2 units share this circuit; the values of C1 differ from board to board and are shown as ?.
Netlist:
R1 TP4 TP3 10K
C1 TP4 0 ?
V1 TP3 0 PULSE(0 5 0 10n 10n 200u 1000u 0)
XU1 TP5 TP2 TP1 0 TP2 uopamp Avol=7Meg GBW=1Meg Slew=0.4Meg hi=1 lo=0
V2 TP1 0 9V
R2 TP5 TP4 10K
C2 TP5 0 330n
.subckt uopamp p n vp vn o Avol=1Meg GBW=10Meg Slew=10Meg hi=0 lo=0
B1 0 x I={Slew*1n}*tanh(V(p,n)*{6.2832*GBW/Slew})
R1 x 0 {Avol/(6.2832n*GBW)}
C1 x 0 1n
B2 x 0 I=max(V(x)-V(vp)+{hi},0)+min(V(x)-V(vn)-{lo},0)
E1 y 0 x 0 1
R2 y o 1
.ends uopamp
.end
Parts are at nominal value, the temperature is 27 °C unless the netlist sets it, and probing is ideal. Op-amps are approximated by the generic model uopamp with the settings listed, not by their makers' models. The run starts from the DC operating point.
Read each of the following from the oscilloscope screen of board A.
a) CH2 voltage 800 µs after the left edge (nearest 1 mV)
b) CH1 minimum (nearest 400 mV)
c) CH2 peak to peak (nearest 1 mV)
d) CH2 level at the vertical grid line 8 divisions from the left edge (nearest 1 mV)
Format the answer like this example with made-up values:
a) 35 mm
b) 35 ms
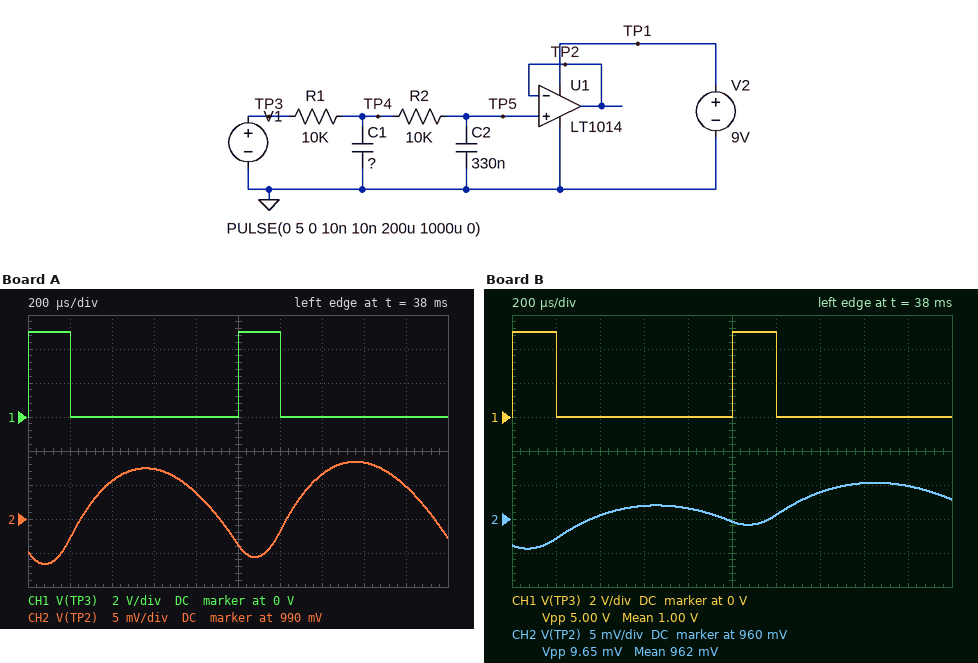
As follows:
a) 994 mV
b) 0 V
c) 15 mV
d) 998 mV
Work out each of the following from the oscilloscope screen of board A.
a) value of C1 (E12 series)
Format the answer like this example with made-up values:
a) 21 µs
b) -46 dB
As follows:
a) 220 nF
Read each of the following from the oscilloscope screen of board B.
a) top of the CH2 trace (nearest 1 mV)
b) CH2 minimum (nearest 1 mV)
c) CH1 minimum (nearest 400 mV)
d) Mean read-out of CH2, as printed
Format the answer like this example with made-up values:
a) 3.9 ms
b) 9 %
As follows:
a) 965 mV
b) 956 mV
c) 0 V
d) 962 mV
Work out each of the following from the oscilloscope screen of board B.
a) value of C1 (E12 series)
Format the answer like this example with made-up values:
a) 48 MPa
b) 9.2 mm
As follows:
a) 680 nF
